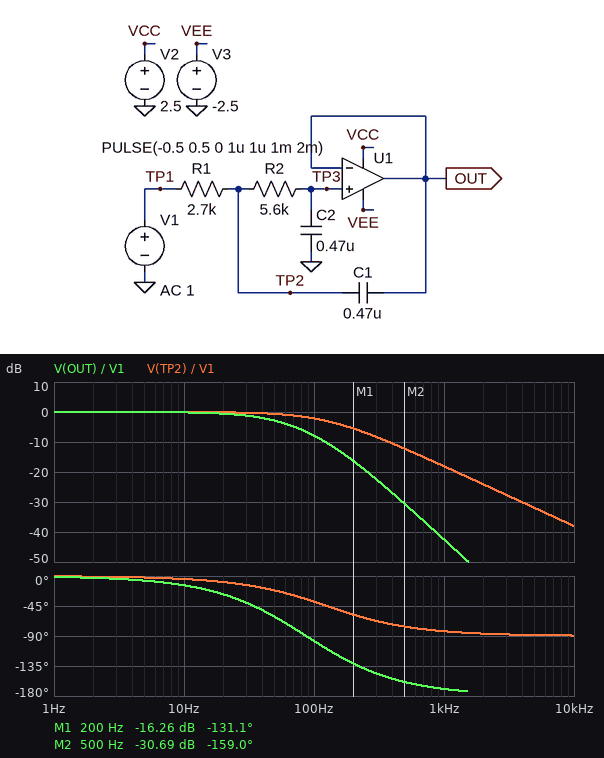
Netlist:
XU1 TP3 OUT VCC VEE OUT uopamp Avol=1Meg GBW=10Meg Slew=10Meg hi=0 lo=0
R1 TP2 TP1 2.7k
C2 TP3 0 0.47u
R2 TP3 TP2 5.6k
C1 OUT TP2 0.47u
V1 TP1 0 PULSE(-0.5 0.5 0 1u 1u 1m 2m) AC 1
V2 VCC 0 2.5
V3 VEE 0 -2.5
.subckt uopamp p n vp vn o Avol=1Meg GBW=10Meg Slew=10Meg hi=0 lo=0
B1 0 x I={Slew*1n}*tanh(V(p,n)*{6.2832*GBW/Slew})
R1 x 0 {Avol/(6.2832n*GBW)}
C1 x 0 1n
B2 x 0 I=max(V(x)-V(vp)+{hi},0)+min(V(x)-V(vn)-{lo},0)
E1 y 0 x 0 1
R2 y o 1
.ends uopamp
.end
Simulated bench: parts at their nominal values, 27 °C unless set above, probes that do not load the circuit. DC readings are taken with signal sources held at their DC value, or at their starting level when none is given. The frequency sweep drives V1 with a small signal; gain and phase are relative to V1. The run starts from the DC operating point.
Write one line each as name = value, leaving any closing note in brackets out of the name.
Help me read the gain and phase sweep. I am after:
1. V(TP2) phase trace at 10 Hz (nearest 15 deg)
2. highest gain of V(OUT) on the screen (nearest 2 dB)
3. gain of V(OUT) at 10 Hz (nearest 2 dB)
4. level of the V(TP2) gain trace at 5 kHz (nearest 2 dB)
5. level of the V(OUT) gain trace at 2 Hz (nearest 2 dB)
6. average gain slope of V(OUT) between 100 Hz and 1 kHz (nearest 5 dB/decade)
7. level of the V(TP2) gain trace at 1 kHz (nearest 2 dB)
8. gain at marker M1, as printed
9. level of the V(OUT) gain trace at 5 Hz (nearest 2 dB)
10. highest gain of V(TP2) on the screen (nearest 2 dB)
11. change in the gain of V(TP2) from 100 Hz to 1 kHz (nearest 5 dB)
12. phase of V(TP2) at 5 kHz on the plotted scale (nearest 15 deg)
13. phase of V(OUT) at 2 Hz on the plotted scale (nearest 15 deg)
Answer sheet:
V(TP2) phase trace at 10 Hz = 0 deg
highest gain of V(OUT) on the screen = 0 dB
gain of V(OUT) at 10 Hz = 0 dB
level of the V(TP2) gain trace at 5 kHz = -32 dB
level of the V(OUT) gain trace at 2 Hz = 0 dB
average gain slope of V(OUT) between 100 Hz and 1 kHz = -35 dB/decade
level of the V(TP2) gain trace at 1 kHz = -18 dB
gain at marker M1, as printed = -16.26 dB
level of the V(OUT) gain trace at 5 Hz = 0 dB
highest gain of V(TP2) on the screen = 0 dB
change in the gain of V(TP2) from 100 Hz to 1 kHz = -15 dB
phase of V(TP2) at 5 kHz on the plotted scale = -90 deg
phase of V(OUT) at 2 Hz on the plotted scale = 0 deg
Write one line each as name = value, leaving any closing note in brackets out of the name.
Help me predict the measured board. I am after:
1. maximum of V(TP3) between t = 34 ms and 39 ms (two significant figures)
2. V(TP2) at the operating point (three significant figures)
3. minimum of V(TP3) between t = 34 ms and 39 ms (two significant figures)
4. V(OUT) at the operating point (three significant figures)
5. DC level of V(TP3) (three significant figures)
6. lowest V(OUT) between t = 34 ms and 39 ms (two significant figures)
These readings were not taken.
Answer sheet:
maximum of V(TP3) between t = 34 ms and 39 ms = 19 mV
V(TP2) at the operating point = -500 mV
minimum of V(TP3) between t = 34 ms and 39 ms = -18 mV
V(OUT) at the operating point = -500 mV
DC level of V(TP3) = -500 mV
lowest V(OUT) between t = 34 ms and 39 ms = -18 mV
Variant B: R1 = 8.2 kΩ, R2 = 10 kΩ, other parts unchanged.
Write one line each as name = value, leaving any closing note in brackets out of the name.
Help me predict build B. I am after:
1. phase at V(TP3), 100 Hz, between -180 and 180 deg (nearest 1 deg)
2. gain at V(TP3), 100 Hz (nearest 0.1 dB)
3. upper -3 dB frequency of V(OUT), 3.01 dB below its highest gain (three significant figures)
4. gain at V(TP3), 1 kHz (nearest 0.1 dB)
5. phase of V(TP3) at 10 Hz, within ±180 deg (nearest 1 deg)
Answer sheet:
phase at V(TP3), 100 Hz, between -180 and 180 deg = -139 deg
gain at V(TP3), 100 Hz = -18.2 dB
upper -3 dB frequency of V(OUT), 3.01 dB below its highest gain = 23.9 Hz
gain at V(TP3), 1 kHz = -57.1 dB
phase of V(TP3) at 10 Hz, within ±180 deg = -30 deg
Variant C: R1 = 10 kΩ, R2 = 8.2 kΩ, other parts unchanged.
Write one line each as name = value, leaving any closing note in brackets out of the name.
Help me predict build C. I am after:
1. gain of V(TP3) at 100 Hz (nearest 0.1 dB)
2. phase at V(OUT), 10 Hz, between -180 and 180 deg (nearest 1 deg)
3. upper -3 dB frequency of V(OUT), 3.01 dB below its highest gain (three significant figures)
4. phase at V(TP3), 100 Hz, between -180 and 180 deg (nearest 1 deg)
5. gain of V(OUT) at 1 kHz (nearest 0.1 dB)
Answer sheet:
gain of V(TP3) at 100 Hz = -18.2 dB
phase at V(OUT), 10 Hz, between -180 and 180 deg = -30 deg
upper -3 dB frequency of V(OUT), 3.01 dB below its highest gain = 23.9 Hz
phase at V(TP3), 100 Hz, between -180 and 180 deg = -139 deg
gain of V(OUT) at 1 kHz = -57.1 dB
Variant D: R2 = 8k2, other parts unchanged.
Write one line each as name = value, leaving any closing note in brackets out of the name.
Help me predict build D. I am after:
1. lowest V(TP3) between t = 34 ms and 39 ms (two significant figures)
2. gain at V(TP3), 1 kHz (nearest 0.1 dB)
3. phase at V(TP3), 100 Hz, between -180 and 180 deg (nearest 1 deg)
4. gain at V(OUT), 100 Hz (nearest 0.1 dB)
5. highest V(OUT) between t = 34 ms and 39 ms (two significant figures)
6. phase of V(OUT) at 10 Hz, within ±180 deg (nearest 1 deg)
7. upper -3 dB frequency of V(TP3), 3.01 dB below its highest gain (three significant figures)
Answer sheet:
lowest V(TP3) between t = 34 ms and 39 ms = -12 mV
gain at V(TP3), 1 kHz = -45.8 dB
phase at V(TP3), 100 Hz, between -180 and 180 deg = -106 deg
gain at V(OUT), 100 Hz = -10.5 dB
highest V(OUT) between t = 34 ms and 39 ms = 13 mV
phase of V(OUT) at 10 Hz, within ±180 deg = -18 deg
upper -3 dB frequency of V(TP3), 3.01 dB below its highest gain = 37.7 Hz
